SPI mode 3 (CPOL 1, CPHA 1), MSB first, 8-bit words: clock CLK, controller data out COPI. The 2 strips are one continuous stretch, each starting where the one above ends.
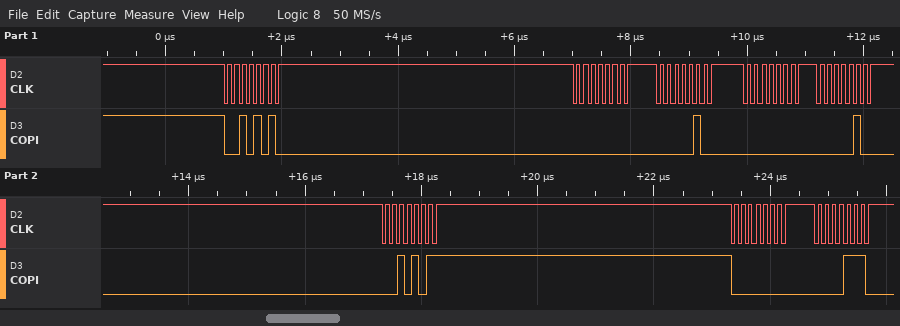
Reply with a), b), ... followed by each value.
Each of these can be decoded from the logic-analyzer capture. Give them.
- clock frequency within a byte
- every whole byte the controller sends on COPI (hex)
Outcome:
a) 8 MHz
b) 0x2A 0x00 0x04 0x00 0x04 0x2B 0x00 0x0E
